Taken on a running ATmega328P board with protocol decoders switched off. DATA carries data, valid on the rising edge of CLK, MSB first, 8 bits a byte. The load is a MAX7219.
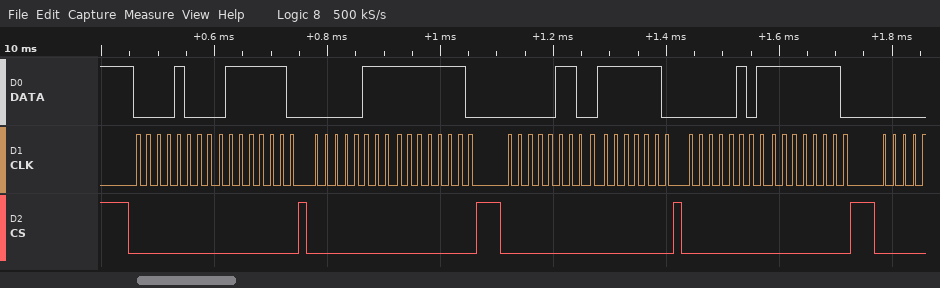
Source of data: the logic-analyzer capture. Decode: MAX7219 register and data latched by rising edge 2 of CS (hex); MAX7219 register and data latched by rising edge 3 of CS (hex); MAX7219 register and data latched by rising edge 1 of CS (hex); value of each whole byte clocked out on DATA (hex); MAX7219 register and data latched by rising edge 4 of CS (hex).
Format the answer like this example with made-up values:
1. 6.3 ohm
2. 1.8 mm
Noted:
1. register 0x7, data 0xFE
2. register 0x6, data 0x7E
3. register 0x8, data 0x7E
4. 08 7E 07 FE 06 7E 05 FE
5. register 0x5, data 0xFE
